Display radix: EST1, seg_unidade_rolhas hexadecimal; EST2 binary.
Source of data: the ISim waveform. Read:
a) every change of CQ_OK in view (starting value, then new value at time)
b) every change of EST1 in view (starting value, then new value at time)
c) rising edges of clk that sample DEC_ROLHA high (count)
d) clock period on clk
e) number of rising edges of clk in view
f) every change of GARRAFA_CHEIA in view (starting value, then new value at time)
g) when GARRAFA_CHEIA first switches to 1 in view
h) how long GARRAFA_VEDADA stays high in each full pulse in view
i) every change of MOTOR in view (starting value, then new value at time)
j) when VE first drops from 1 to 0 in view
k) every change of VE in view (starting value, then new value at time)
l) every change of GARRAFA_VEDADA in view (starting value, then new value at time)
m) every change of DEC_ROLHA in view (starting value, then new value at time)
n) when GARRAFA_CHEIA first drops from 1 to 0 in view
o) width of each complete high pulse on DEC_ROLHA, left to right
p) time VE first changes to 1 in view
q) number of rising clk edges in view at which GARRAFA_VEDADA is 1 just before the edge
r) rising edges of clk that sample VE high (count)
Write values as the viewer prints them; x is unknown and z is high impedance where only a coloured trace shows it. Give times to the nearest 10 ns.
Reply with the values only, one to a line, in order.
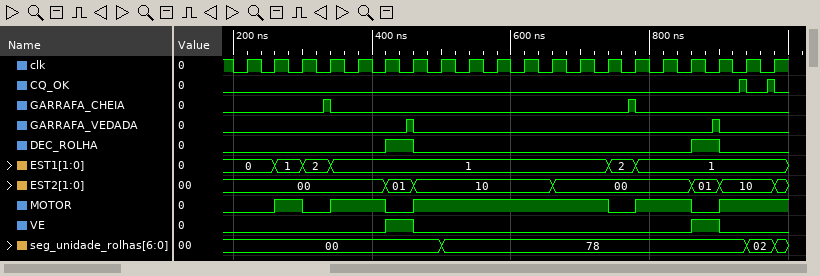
0, 1 at 930 ns, 0 at 940 ns, 1 at 970 ns, 0 at 980 ns
0, 1 at 260 ns, 2 at 300 ns, 1 at 340 ns, 2 at 740 ns, 1 at 780 ns
2
40 ns
20
0, 1 at 330 ns, 0 at 340 ns, 1 at 770 ns, 0 at 780 ns
330 ns
10 ns, 10 ns
0, 1 at 260 ns, 0 at 300 ns, 1 at 340 ns, 0 at 420 ns, 1 at 460 ns, 0 at 740 ns, 1 at 780 ns, 0 at 860 ns, 1 at 900 ns
460 ns
0, 1 at 420 ns, 0 at 460 ns, 1 at 860 ns, 0 at 900 ns
0, 1 at 450 ns, 0 at 460 ns, 1 at 890 ns, 0 at 900 ns
0, 1 at 420 ns, 0 at 460 ns, 1 at 860 ns, 0 at 900 ns
340 ns
40 ns, 40 ns
420 ns
2
2
